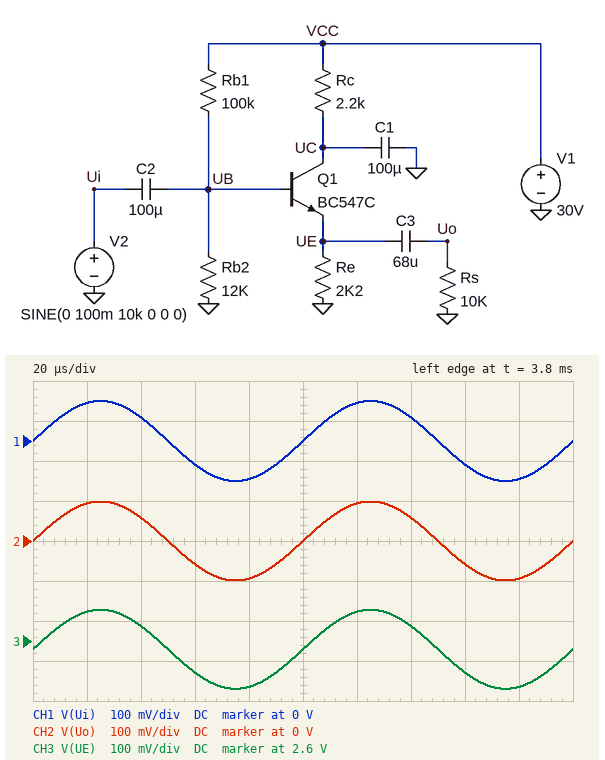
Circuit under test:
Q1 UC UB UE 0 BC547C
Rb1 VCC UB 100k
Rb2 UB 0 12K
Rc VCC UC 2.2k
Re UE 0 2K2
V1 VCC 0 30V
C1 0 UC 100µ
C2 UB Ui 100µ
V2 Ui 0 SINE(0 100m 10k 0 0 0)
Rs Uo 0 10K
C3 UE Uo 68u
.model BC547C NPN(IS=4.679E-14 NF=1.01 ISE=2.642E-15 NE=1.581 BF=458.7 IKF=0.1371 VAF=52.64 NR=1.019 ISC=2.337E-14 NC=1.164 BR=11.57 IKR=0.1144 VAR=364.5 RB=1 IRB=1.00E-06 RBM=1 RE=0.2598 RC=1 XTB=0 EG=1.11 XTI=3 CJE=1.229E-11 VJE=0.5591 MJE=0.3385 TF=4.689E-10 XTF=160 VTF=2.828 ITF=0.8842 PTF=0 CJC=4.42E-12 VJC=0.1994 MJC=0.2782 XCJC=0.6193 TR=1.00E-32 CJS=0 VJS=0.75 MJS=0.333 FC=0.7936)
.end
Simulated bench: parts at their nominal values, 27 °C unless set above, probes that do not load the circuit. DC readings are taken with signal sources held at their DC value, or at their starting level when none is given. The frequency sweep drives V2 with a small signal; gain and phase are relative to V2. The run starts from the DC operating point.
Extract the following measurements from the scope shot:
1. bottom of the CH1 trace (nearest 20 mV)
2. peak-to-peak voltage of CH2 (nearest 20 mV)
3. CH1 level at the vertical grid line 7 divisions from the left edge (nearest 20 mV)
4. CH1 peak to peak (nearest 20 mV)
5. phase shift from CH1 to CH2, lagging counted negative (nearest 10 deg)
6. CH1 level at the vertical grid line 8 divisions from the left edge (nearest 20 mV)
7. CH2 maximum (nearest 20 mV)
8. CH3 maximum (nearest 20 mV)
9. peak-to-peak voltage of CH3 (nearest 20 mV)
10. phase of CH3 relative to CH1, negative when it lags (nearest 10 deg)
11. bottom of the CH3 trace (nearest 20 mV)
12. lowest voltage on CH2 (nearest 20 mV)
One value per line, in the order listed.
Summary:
-100 mV
200 mV
60 mV
200 mV
0 deg
-60 mV
100 mV
2.68 V
200 mV
0 deg
2.48 V
-100 mV
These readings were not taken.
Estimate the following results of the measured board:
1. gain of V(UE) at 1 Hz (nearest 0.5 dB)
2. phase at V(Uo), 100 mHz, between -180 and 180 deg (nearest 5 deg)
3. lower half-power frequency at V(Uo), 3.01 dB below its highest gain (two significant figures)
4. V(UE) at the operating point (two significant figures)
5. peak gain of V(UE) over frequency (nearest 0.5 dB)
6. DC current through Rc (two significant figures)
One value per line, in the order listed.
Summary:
0 dB
125 deg
300 mHz
2.6 V
0 dB
1.2 mA
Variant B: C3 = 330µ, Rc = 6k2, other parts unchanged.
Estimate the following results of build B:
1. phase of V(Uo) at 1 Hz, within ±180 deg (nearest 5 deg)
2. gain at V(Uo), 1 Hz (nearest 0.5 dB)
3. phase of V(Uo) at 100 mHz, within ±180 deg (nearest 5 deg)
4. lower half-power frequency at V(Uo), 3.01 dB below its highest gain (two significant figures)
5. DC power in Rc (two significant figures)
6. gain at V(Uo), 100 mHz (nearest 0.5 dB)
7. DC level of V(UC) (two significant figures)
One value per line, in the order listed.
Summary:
10 deg
0 dB
80 deg
160 mHz
8.5 mW
-6.0 dB
23 V
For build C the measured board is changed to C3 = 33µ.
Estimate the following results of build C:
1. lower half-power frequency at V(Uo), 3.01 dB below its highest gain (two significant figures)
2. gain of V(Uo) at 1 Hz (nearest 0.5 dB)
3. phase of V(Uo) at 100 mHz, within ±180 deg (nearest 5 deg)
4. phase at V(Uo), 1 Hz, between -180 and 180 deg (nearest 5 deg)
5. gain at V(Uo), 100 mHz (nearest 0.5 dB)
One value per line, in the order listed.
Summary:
520 mHz
-1.0 dB
135 deg
35 deg
-19.0 dB
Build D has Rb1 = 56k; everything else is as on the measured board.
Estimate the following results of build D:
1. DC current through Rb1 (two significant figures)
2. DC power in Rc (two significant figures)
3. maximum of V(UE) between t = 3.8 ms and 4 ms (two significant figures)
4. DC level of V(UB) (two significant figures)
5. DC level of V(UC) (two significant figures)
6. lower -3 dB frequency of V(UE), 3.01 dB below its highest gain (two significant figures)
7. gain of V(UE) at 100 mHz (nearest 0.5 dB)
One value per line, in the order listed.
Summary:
440 µA
9.7 mW
4.7 V
5.3 V
25 V
160 mHz
-5.5 dB
